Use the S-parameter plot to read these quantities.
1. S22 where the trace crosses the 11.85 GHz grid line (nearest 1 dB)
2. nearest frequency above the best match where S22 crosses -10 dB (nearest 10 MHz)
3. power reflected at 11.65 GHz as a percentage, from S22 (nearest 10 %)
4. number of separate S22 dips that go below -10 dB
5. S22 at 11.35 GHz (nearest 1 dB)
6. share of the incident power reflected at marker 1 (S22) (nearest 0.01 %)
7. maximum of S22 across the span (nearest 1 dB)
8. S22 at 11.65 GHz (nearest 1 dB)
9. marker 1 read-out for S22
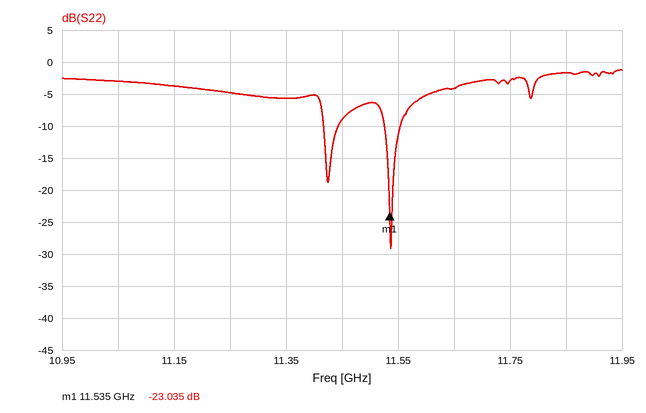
-2 dB
11.55 GHz
40 %
2
-6 dB
0.50 %
-1 dB
-4 dB
-23.035 dB
